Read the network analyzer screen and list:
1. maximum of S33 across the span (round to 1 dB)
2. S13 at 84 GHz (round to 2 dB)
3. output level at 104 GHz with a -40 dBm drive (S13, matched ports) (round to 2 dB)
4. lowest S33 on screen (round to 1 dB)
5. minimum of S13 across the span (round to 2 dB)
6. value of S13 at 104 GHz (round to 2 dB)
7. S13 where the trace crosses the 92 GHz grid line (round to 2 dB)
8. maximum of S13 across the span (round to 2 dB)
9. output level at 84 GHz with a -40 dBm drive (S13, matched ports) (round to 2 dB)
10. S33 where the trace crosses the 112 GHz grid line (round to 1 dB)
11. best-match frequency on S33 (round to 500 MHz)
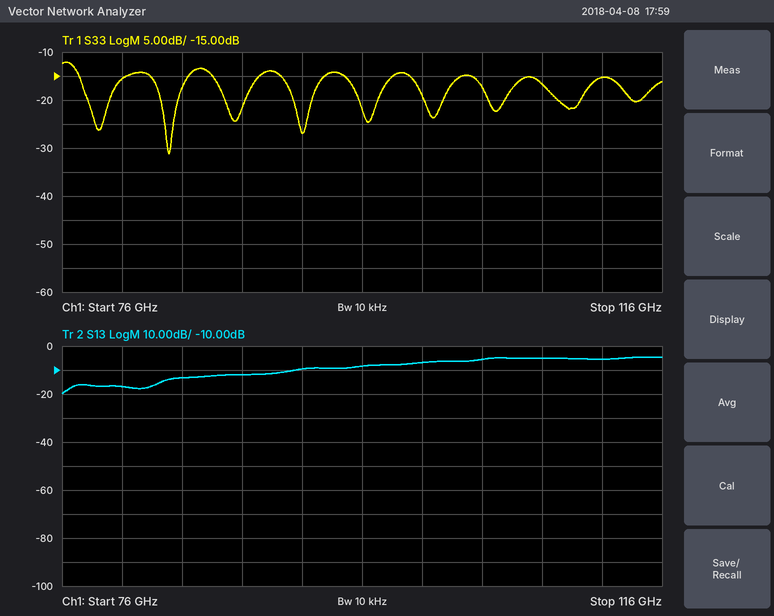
-12 dB
-14 dB
-46 dBm
-31 dB
-20 dB
-6 dB
-10 dB
-4 dB
-54 dBm
-15 dB
83.0 GHz
